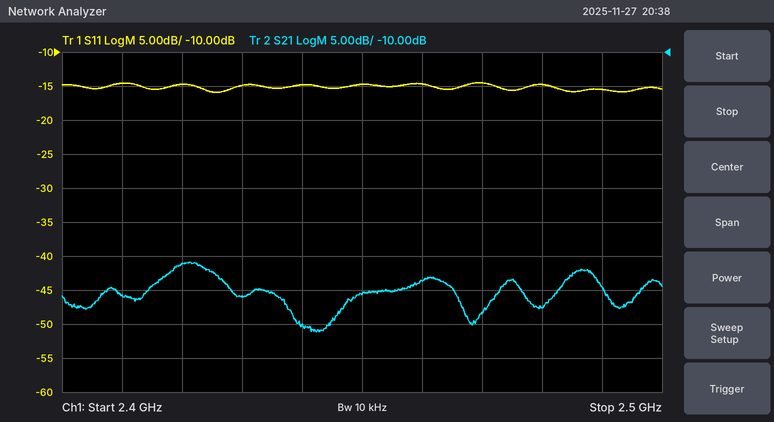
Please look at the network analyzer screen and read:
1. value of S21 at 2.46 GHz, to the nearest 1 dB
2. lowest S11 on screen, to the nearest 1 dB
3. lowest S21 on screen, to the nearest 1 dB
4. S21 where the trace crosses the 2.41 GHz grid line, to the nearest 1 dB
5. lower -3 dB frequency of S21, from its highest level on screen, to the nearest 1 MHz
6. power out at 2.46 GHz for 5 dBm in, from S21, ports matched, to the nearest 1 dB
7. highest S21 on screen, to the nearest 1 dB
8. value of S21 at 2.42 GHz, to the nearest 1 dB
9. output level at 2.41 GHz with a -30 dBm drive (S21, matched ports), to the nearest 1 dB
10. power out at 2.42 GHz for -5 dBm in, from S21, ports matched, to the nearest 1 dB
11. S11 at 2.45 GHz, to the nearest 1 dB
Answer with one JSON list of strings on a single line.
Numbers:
["-44 dB", "-16 dB", "-51 dB", "-46 dB", "2.416 GHz", "-39 dBm", "-41 dB", "-41 dB", "-76 dBm", "-46 dBm", "-15 dB"]
